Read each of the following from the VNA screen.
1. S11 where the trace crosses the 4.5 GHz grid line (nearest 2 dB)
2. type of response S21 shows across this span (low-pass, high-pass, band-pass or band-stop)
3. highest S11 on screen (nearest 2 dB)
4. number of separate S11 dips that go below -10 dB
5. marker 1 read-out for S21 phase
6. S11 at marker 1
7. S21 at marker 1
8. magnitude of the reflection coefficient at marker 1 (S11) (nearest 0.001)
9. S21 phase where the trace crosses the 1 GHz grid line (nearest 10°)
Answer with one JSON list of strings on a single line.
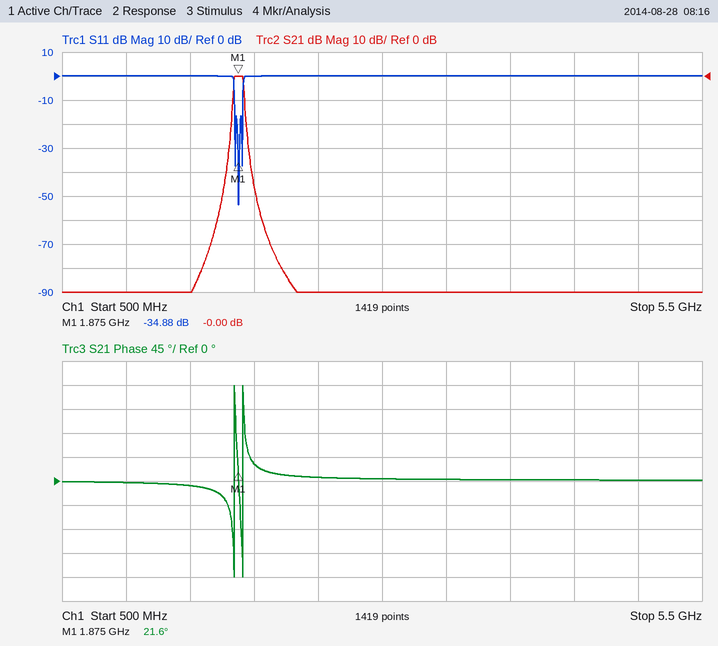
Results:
["0 dB", "band-pass", "0 dB", "3", "21.6°", "-34.88 dB", "-0.00 dB", "0.018", "0°"]
